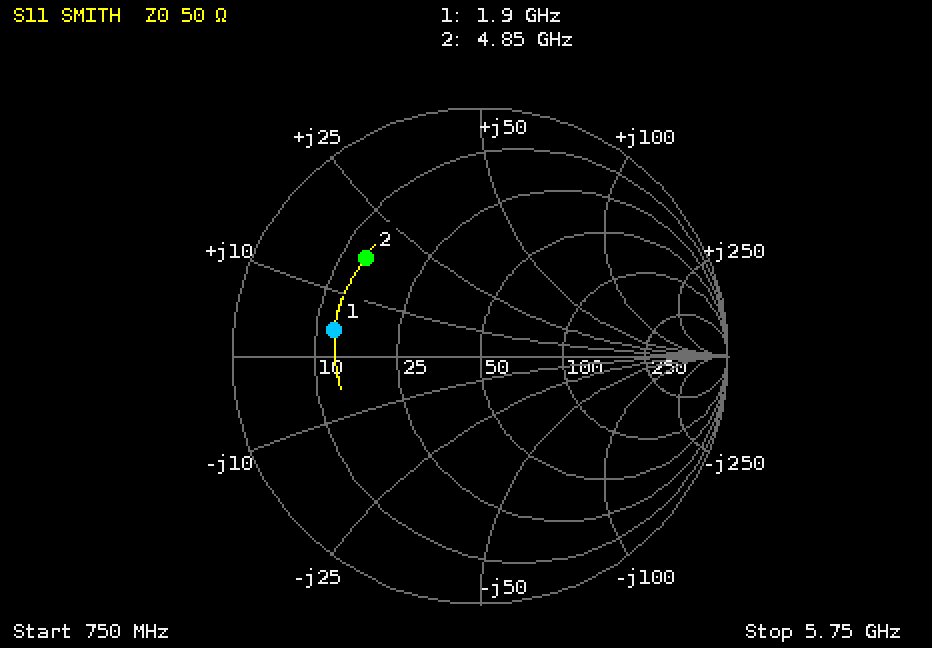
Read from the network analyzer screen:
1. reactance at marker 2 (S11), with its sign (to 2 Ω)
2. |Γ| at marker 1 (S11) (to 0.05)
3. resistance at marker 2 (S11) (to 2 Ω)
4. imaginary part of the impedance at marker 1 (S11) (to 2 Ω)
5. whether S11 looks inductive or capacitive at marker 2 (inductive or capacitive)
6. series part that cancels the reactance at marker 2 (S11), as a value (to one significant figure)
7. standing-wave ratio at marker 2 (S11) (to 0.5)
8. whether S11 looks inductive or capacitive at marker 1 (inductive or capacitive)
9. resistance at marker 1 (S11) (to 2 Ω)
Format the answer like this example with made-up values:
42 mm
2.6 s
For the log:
+18 Ω
0.60
14 Ω
+4 Ω
inductive
2 pF
4.0
inductive
12 Ω
